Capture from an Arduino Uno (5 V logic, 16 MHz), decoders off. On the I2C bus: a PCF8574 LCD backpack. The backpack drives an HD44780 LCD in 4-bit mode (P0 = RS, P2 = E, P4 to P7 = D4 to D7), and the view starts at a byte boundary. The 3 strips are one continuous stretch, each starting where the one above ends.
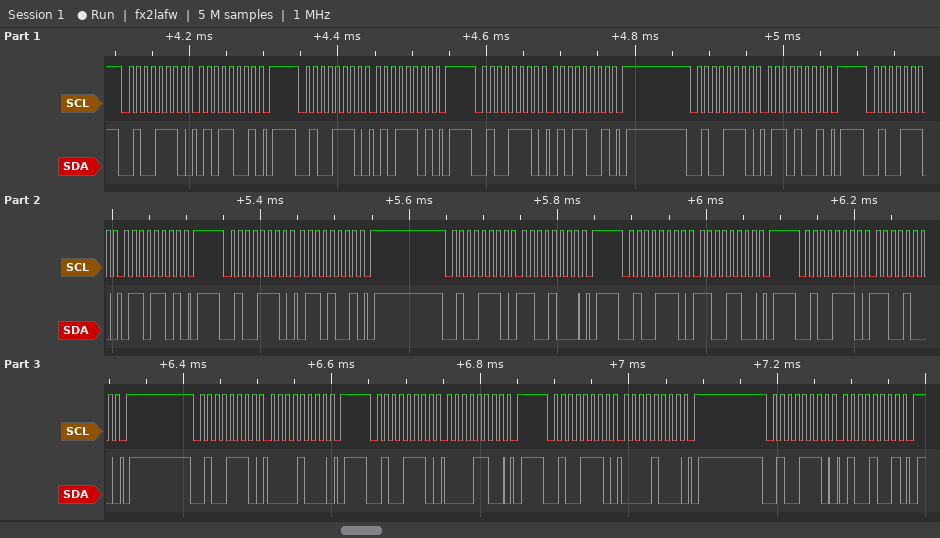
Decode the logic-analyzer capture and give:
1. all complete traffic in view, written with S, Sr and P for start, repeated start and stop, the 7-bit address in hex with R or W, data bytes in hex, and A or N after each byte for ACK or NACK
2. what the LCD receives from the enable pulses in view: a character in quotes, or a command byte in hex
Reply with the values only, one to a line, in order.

S 27W A 59 A P S 27W A 5D A P S 27W A 59 A P S 27W A 69 A P S 27W A 6D A P S 27W A 69 A P S 27W A C8 A P S 27W A CC A P S 27W A C8 A P S 27W A 08 A P S 27W A 0C A P S 27W A 08 A P S 27W A 49 A P
'V' 0xC0
